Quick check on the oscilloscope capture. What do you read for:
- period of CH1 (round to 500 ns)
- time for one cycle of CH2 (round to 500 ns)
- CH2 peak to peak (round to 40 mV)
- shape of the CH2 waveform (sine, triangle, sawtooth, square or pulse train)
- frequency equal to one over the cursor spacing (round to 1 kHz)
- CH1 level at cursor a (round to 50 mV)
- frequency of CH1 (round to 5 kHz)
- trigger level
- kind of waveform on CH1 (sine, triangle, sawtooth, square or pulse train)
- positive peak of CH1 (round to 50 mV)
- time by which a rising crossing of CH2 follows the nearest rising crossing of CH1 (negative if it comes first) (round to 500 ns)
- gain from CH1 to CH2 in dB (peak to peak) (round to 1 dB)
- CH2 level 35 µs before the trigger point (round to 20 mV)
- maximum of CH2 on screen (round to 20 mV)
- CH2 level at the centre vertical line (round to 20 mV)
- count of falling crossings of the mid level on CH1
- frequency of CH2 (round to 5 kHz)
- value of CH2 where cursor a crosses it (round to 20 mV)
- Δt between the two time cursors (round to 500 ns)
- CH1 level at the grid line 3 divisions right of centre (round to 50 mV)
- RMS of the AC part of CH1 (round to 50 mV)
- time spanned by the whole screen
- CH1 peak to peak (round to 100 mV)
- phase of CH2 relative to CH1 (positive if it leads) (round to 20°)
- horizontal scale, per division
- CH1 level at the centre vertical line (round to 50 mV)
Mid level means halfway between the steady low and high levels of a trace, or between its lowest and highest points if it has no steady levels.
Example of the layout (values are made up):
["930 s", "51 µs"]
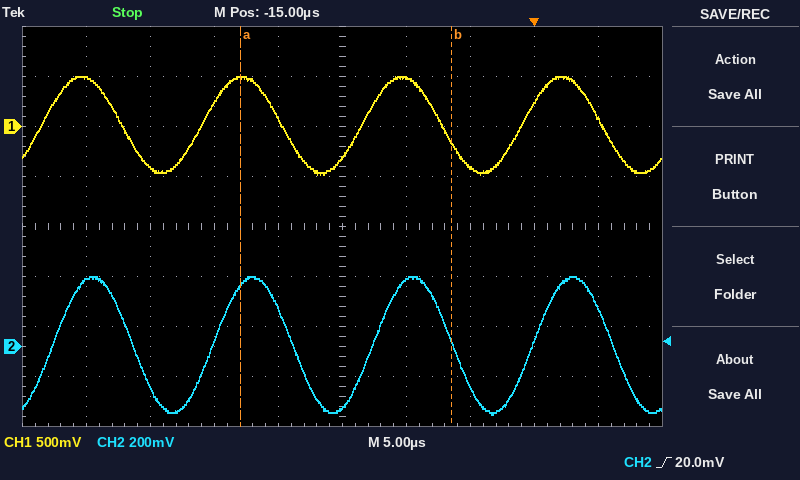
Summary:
["12.5 µs", "12.5 µs", "560 mV", "sine", "61 kHz", "500 mV", "80 kHz", "20.0 mV", "sine", "500 mV", "+1.0 µs", "-5 dB", "260 mV", "280 mV", "-240 mV", "4", "80 kHz", "240 mV", "16.5 µs", "250 mV", "350 mV", "50 µs", "1.00 V", "-20°", "5 µs", "-300 mV"]
